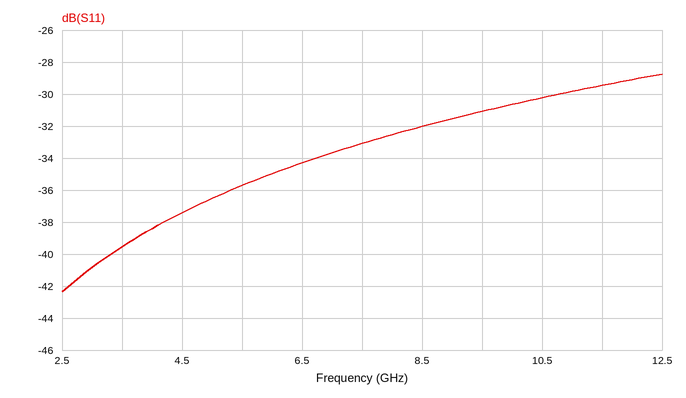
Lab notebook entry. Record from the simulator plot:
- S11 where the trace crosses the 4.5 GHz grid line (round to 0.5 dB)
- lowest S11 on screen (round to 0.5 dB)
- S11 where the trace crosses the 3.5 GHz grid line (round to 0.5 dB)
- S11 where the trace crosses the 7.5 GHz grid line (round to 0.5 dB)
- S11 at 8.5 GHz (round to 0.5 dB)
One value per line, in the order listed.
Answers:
-37.5 dB
-42.5 dB
-39.5 dB
-33.0 dB
-32.0 dB
